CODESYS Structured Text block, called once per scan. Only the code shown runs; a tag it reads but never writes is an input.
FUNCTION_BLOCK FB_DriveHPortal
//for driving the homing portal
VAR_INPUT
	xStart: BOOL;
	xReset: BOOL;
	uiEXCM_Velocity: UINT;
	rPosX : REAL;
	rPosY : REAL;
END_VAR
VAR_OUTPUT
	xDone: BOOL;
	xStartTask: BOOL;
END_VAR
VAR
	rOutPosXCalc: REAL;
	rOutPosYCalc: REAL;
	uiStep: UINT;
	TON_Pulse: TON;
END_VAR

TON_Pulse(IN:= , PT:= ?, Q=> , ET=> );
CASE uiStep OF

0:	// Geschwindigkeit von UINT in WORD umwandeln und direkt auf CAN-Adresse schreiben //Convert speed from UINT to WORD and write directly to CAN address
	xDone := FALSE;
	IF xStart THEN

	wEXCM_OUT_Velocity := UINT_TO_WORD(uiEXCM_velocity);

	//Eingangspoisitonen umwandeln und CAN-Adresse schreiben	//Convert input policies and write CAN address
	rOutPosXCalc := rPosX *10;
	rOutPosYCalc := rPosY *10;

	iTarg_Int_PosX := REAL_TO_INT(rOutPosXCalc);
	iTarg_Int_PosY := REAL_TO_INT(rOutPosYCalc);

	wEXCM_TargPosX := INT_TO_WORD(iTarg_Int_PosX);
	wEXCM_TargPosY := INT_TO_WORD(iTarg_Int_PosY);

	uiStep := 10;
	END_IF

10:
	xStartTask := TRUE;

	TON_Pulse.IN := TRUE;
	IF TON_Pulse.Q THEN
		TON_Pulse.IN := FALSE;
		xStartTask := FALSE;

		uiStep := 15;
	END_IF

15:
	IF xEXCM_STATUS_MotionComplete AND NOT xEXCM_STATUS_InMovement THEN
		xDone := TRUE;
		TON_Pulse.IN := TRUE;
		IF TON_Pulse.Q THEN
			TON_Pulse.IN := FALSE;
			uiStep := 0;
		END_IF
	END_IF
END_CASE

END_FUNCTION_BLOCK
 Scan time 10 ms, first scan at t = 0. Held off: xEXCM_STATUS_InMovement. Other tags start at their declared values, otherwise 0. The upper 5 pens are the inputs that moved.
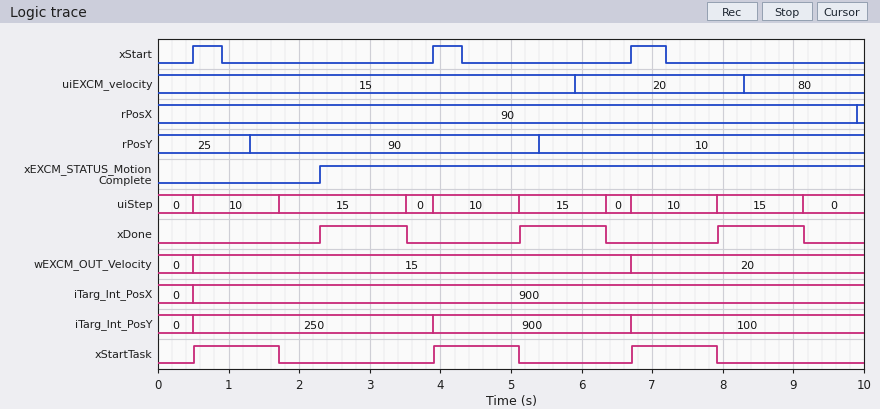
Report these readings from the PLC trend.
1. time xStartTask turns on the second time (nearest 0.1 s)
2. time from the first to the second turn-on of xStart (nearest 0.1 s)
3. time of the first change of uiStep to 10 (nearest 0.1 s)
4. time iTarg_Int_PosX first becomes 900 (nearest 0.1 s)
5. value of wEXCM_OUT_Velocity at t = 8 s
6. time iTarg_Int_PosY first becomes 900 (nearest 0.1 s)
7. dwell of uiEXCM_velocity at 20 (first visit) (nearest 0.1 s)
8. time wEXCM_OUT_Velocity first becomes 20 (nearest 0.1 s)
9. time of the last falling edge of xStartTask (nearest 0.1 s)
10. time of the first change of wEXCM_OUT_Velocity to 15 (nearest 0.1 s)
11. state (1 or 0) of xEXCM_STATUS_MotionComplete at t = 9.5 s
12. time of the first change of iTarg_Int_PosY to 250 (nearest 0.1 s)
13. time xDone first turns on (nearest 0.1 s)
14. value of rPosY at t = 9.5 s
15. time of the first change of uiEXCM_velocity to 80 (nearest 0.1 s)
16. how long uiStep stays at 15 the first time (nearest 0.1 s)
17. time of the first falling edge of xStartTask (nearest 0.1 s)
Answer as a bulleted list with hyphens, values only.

- 3.9 s
- 3.4 s
- 0.5 s
- 0.5 s
- 20
- 3.9 s
- 2.4 s
- 6.7 s
- 7.9 s
- 0.5 s
- 1
- 0.5 s
- 2.3 s
- 10
- 8.3 s
- 1.8 s
- 1.7 s
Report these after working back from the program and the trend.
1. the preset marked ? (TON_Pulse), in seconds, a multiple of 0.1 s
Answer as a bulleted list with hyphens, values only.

- 1.2 s
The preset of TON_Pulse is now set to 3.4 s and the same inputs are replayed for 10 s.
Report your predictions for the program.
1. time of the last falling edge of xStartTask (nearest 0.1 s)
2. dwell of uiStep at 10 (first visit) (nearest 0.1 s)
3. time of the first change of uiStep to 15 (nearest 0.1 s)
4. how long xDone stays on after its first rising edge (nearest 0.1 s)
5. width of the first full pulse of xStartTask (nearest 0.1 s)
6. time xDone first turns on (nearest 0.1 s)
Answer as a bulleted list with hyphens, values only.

- 3.9 s
- 3.4 s
- 3.9 s
- 3.4 s
- 3.4 s
- 3.9 s
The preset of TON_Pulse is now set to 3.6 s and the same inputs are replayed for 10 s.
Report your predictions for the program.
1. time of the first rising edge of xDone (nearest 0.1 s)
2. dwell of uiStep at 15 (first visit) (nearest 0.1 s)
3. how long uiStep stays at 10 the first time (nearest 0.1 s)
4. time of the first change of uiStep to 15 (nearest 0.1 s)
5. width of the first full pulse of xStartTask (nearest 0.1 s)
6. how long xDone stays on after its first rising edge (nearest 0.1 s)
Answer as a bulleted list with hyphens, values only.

- 4.1 s
- 3.6 s
- 3.6 s
- 4.1 s
- 3.6 s
- 3.6 s
